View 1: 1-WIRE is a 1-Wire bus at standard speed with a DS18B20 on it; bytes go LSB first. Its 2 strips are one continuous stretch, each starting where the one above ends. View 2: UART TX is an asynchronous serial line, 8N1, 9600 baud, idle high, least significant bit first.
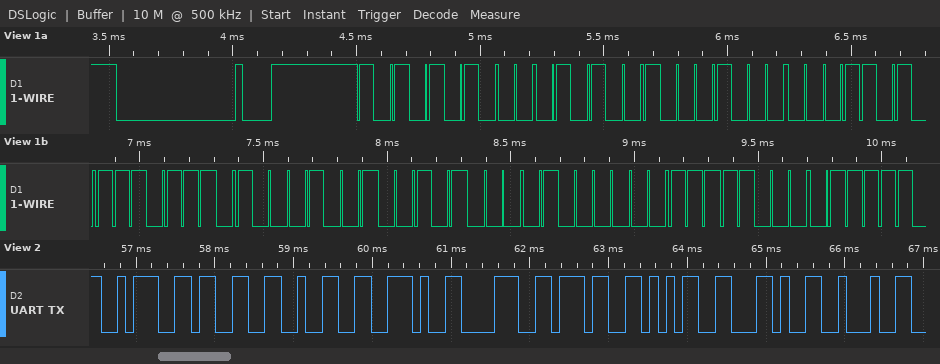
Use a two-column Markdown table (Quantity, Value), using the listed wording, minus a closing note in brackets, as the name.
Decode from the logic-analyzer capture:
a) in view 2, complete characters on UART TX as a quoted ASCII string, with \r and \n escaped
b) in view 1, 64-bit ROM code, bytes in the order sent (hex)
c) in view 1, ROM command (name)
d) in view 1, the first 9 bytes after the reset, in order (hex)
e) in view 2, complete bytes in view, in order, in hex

| Quantity | Value |
|---|---|
| in view 2, complete characters on UART TX as a quoted ASCII string, with \r and \n escaped | ":32.875,\"" |
| in view 1, 64-bit ROM code, bytes in the order sent | 28 11 58 77 91 14 02 1F |
| in view 1, ROM command | Match ROM |
| in view 1, the first 9 bytes after the reset, in order | 55 28 11 58 77 91 14 02 1F |
| in view 2, complete bytes in view, in order, in hex | 3A 33 32 2E 38 37 35 2C 22 |
